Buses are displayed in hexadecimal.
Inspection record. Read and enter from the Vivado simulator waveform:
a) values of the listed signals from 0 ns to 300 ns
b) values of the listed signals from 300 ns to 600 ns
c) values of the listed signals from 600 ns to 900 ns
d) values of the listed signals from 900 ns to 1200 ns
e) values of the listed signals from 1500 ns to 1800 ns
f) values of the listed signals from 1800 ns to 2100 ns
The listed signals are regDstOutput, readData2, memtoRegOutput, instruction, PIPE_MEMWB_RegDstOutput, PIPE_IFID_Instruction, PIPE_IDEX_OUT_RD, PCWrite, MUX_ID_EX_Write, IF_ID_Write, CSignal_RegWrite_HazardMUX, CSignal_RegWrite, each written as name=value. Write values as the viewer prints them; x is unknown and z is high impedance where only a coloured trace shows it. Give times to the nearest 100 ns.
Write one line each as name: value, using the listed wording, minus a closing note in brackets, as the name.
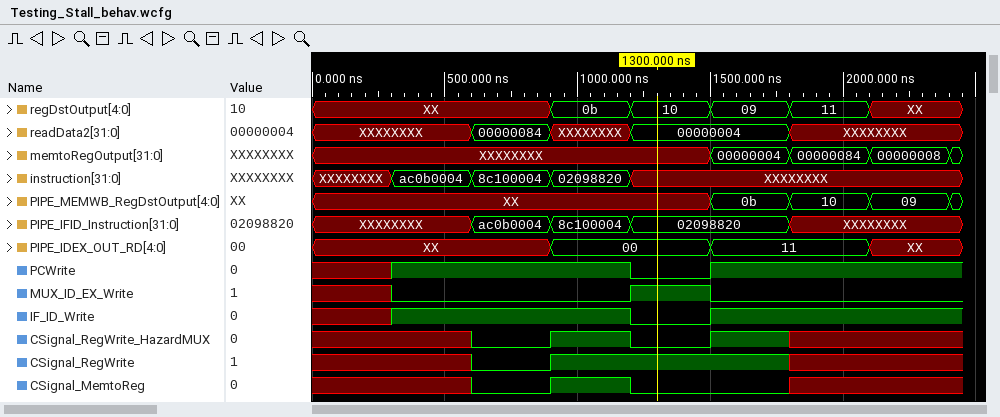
values of the listed signals from 0 ns to 300 ns: regDstOutput=XX, readData2=XXXXXXXX, memtoRegOutput=XXXXXXXX, instruction=XXXXXXXX, PIPE_MEMWB_RegDstOutput=XX, PIPE_IFID_Instruction=XXXXXXXX, PIPE_IDEX_OUT_RD=XX, PCWrite=x, MUX_ID_EX_Write=x, IF_ID_Write=x, CSignal_RegWrite_HazardMUX=x, CSignal_RegWrite=x
values of the listed signals from 300 ns to 600 ns: regDstOutput=XX, readData2=XXXXXXXX, memtoRegOutput=XXXXXXXX, instruction=ac0b0004, PIPE_MEMWB_RegDstOutput=XX, PIPE_IFID_Instruction=XXXXXXXX, PIPE_IDEX_OUT_RD=XX, PCWrite=1, MUX_ID_EX_Write=0, IF_ID_Write=1, CSignal_RegWrite_HazardMUX=x, CSignal_RegWrite=x
values of the listed signals from 600 ns to 900 ns: regDstOutput=XX, readData2=00000084, memtoRegOutput=XXXXXXXX, instruction=8c100004, PIPE_MEMWB_RegDstOutput=XX, PIPE_IFID_Instruction=ac0b0004, PIPE_IDEX_OUT_RD=XX, PCWrite=1, MUX_ID_EX_Write=0, IF_ID_Write=1, CSignal_RegWrite_HazardMUX=0, CSignal_RegWrite=0
values of the listed signals from 900 ns to 1200 ns: regDstOutput=0b, readData2=XXXXXXXX, memtoRegOutput=XXXXXXXX, instruction=02098820, PIPE_MEMWB_RegDstOutput=XX, PIPE_IFID_Instruction=8c100004, PIPE_IDEX_OUT_RD=00, PCWrite=1, MUX_ID_EX_Write=0, IF_ID_Write=1, CSignal_RegWrite_HazardMUX=1, CSignal_RegWrite=1
values of the listed signals from 1500 ns to 1800 ns: regDstOutput=09, readData2=00000004, memtoRegOutput=00000004, instruction=XXXXXXXX, PIPE_MEMWB_RegDstOutput=0b, PIPE_IFID_Instruction=02098820, PIPE_IDEX_OUT_RD=11, PCWrite=1, MUX_ID_EX_Write=0, IF_ID_Write=1, CSignal_RegWrite_HazardMUX=1, CSignal_RegWrite=1
values of the listed signals from 1800 ns to 2100 ns: regDstOutput=11, readData2=XXXXXXXX, memtoRegOutput=00000084, instruction=XXXXXXXX, PIPE_MEMWB_RegDstOutput=10, PIPE_IFID_Instruction=XXXXXXXX, PIPE_IDEX_OUT_RD=11, PCWrite=1, MUX_ID_EX_Write=0, IF_ID_Write=1, CSignal_RegWrite_HazardMUX=x, CSignal_RegWrite=x
